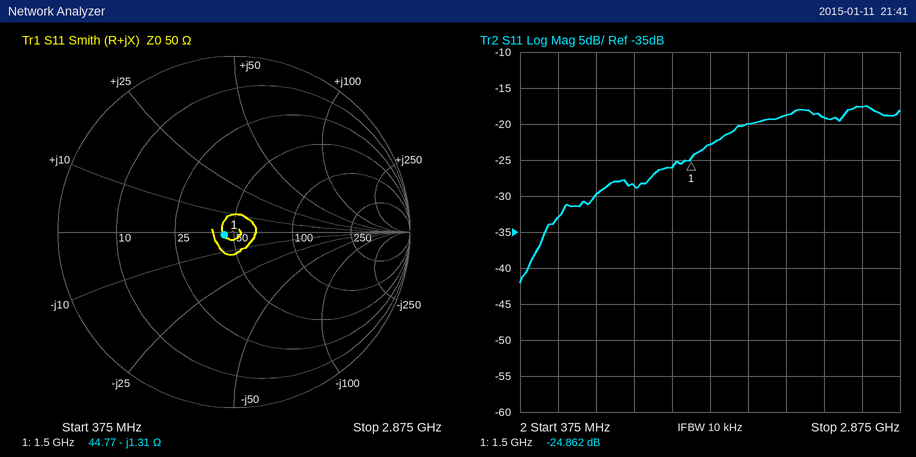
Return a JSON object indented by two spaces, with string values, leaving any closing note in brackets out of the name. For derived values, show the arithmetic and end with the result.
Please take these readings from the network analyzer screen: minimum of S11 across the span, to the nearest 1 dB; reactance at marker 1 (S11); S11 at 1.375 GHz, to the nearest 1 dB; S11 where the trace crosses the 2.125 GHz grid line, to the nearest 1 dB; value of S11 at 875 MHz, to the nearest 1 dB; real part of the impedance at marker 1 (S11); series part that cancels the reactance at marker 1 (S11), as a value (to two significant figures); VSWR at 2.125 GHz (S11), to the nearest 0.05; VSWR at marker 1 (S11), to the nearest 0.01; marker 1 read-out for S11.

{
  "minimum of S11 across the span, to the nearest 1 dB": "-42 dB",
  "reactance at marker 1": "-1.31 Ω",
  "S11 at 1.375 GHz, to the nearest 1 dB": "-26 dB",
  "S11 where the trace crosses the 2.125 GHz grid line, to the nearest 1 dB": "-19 dB",
  "value of S11 at 875 MHz, to the nearest 1 dB": "-30 dB",
  "real part of the impedance at marker 1": "44.77 Ω",
  "series part that cancels the reactance at marker 1 (S11), as a value": "L = 1.31 Ω/(2π × 1.5 GHz) ≈ 139 pH, so 140 pH to two significant figures",
  "VSWR at 2.125 GHz (S11), to the nearest 0.05": "|Γ| = 10^(-19/20) = 0.1122; VSWR = (1 + 0.1122)/(1 − 0.1122) ≈ 1.25",
  "VSWR at marker 1 (S11), to the nearest 0.01": "1.12",
  "marker 1 read-out for S11": "-24.862 dB"
}
